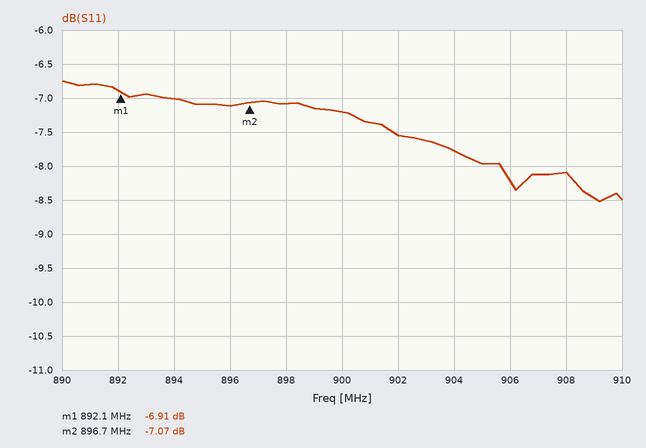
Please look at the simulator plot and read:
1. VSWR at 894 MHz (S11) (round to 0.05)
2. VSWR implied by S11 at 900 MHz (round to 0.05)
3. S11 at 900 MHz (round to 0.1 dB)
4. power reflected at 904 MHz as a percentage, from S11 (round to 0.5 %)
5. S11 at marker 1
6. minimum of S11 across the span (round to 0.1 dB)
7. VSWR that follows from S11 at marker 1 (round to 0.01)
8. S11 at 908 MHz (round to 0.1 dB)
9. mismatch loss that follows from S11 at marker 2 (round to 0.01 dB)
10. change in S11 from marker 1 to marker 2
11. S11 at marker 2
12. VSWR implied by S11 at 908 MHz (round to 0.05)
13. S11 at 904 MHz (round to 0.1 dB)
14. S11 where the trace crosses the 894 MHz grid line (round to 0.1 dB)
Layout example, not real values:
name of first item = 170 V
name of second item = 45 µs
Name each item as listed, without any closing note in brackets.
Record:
VSWR at 894 MHz (S11) = 2.60
VSWR implied by S11 at 900 MHz = 2.55
S11 at 900 MHz = -7.2 dB
power reflected at 904 MHz as a percentage, from S11 = 16.5 %
S11 at marker 1 = -6.91 dB
minimum of S11 across the span = -8.5 dB
VSWR that follows from S11 at marker 1 = 2.65
S11 at 908 MHz = -8.1 dB
mismatch loss that follows from S11 at marker 2 = 0.95 dB
change in S11 from marker 1 to marker 2 = -0.16 dB
S11 at marker 2 = -7.07 dB
VSWR implied by S11 at 908 MHz = 2.30
S11 at 904 MHz = -7.8 dB
S11 where the trace crosses the 894 MHz grid line = -7.0 dB
